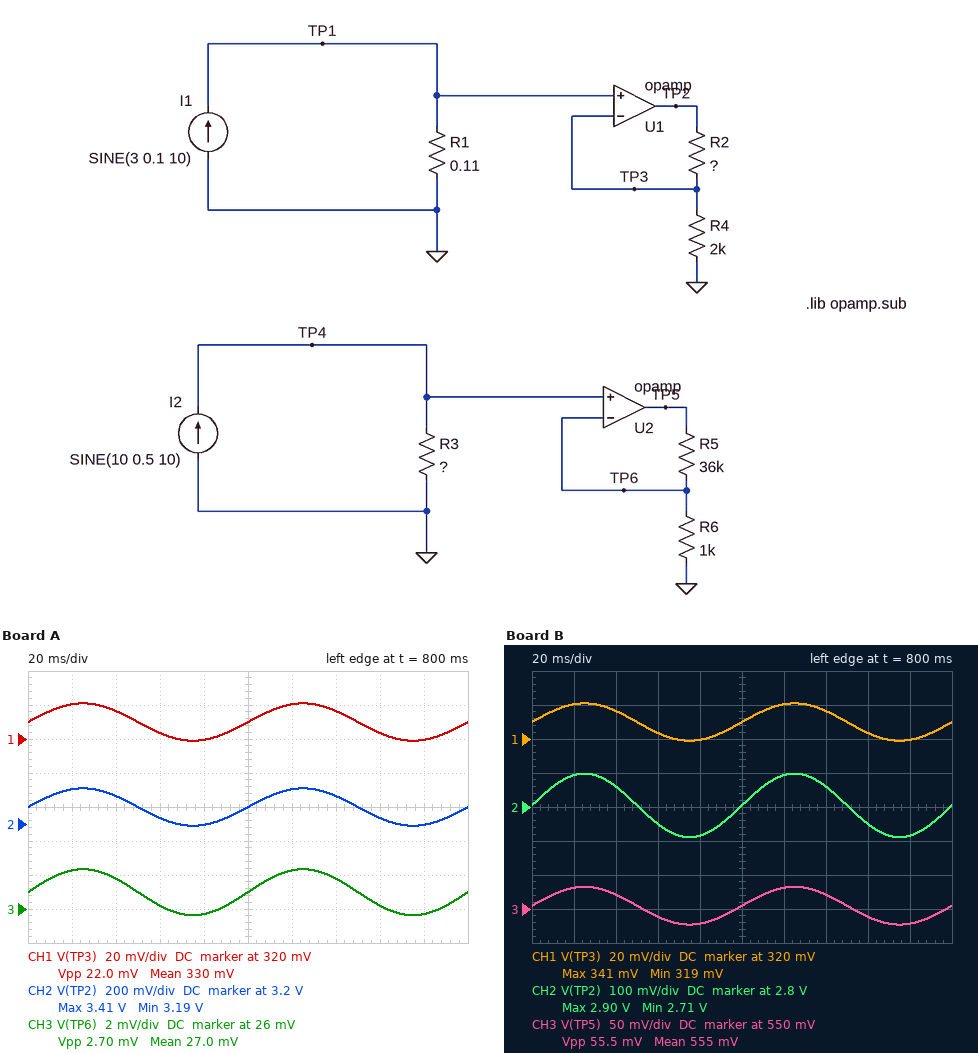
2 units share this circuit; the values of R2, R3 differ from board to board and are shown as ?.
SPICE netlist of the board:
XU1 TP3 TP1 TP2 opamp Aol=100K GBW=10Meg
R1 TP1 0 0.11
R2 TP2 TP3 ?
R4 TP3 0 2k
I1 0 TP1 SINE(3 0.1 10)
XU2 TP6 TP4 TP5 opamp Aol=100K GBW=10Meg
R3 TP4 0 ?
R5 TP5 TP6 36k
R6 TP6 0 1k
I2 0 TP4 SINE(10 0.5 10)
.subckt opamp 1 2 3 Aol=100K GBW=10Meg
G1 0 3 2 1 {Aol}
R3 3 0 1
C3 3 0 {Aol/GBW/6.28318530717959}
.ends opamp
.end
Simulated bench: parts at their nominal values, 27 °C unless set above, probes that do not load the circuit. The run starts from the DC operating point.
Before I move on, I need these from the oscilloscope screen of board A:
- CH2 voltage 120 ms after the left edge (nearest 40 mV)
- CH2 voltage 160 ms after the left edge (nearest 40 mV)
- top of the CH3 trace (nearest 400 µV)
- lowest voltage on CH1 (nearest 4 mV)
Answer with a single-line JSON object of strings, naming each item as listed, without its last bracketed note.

{"CH2 voltage 120 ms after the left edge": "3.40 V", "CH2 voltage 160 ms after the left edge": "3.24 V", "top of the CH3 trace": "28.4 mV", "lowest voltage on CH1": "320 mV"}
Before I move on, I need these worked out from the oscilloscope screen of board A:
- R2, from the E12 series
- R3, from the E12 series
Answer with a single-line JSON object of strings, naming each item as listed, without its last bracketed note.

{"R2, from the E12 series": "18 kΩ", "R3, from the E12 series": "2.7 mΩ"}
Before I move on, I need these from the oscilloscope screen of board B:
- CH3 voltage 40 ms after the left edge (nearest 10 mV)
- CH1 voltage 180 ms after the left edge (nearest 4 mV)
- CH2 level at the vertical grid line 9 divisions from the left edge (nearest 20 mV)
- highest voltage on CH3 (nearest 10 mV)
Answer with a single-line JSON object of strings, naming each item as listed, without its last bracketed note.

{"CH3 voltage 40 ms after the left edge": "570 mV", "CH1 voltage 180 ms after the left edge": "320 mV", "CH2 level at the vertical grid line 9 divisions from the left edge": "2.72 V", "highest voltage on CH3": "580 mV"}
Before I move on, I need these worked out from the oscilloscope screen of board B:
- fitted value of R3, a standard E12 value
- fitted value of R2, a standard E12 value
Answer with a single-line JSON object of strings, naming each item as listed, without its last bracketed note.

{"fitted value of R3, a standard E12 value": "1.5 mΩ", "fitted value of R2, a standard E12 value": "15 kΩ"}
